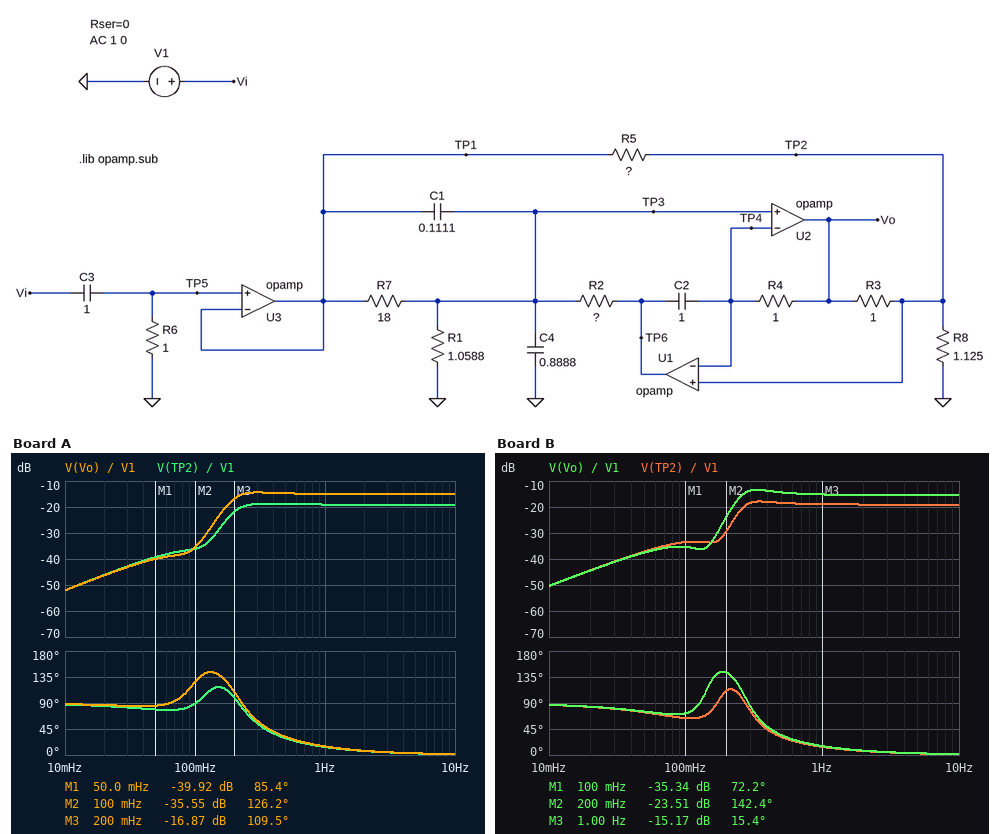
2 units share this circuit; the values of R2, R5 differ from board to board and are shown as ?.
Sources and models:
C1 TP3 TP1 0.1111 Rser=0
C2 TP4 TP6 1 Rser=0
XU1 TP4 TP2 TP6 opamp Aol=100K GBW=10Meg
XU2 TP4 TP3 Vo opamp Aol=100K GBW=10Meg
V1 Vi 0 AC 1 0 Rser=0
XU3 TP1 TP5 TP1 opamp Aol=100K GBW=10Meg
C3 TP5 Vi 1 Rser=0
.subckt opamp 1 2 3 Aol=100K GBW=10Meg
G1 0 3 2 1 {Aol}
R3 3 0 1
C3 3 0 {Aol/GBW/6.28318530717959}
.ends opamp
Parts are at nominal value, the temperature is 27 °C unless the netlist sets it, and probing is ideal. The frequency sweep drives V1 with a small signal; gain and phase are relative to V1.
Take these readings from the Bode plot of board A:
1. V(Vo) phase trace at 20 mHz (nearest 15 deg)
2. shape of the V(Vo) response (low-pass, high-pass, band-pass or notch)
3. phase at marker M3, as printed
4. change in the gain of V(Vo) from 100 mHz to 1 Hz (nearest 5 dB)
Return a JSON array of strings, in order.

["90 deg", "high-pass", "109.5 deg", "20 dB"]
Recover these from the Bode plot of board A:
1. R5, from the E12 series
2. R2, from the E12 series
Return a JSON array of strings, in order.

["27 Ω", "0.56 Ω"]
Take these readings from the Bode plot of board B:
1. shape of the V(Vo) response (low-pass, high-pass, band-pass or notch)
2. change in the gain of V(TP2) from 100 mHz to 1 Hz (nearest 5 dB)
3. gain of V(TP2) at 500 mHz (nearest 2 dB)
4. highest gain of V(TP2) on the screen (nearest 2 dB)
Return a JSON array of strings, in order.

["high-pass", "15 dB", "-18 dB", "-18 dB"]
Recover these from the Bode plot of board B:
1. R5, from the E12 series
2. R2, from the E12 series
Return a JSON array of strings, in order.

["22 Ω", "0.33 Ω"]
